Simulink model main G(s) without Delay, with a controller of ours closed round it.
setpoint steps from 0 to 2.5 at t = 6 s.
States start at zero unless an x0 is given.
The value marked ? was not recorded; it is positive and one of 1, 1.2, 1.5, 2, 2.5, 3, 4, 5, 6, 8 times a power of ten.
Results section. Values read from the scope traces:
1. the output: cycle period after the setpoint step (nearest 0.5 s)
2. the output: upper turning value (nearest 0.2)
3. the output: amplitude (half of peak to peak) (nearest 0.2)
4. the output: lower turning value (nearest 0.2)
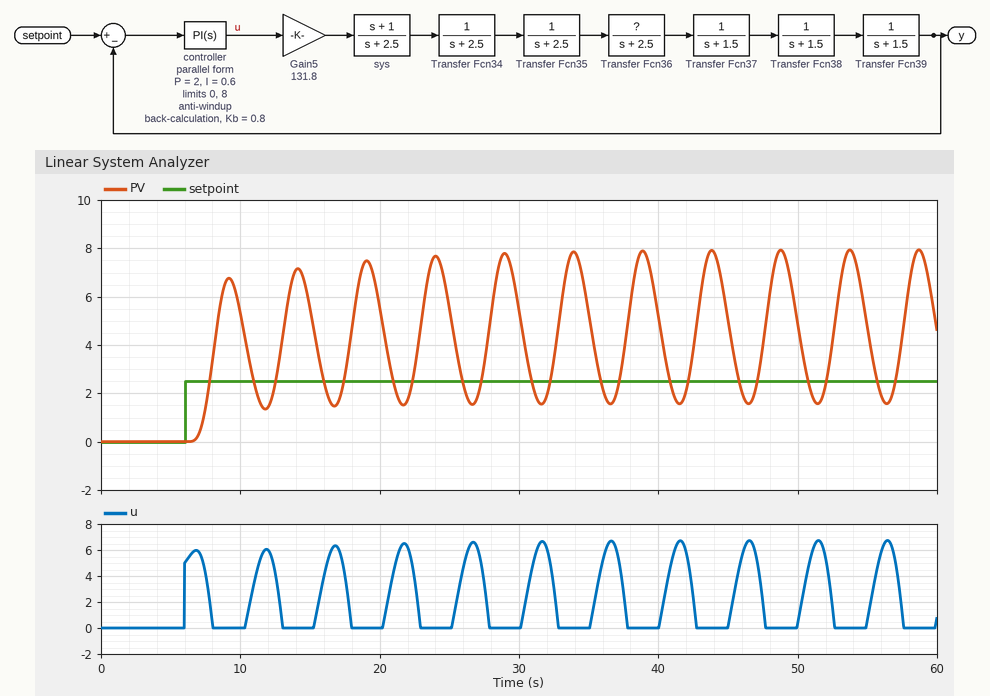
5.0 s
8.0
3.2
1.6
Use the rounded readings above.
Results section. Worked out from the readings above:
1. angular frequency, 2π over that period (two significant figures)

1.3 rad/s
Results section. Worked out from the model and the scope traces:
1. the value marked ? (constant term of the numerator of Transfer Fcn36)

2
